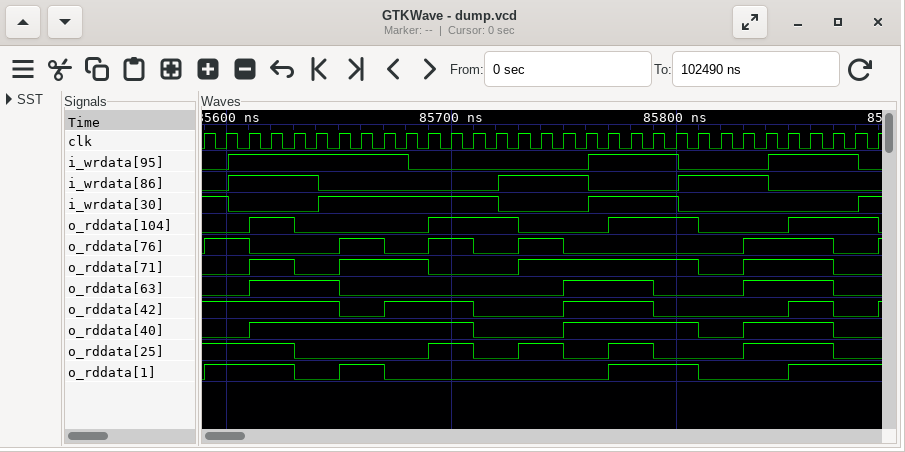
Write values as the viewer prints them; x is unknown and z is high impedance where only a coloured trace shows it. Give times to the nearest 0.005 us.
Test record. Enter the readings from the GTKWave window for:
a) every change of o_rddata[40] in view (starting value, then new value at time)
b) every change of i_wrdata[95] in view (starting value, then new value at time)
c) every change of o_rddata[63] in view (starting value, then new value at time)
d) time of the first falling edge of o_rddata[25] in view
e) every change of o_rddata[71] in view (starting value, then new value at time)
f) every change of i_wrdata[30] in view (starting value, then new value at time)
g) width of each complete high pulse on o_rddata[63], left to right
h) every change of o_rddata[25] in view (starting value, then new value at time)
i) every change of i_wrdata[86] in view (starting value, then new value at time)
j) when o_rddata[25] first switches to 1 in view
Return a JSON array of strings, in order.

["0, 1 at 85.61 us, 0 at 85.71 us, 1 at 85.75 us, 0 at 85.81 us, 1 at 85.83 us, 0 at 85.87 us", "0, 1 at 85.6 us, 0 at 85.68 us, 1 at 85.76 us, 0 at 85.8 us, 1 at 85.84 us, 0 at 85.88 us", "0, 1 at 85.61 us, 0 at 85.65 us, 1 at 85.75 us, 0 at 85.79 us, 1 at 85.83 us, 0 at 85.87 us", "85.63 us", "0, 1 at 85.61 us, 0 at 85.63 us, 1 at 85.65 us, 0 at 85.69 us, 1 at 85.73 us, 0 at 85.81 us, 1 at 85.83 us, 0 at 85.87 us", "1, 0 at 85.6 us, 1 at 85.64 us, 0 at 85.72 us, 1 at 85.76 us, 0 at 85.8 us, 1 at 85.88 us", "0.04 us, 0.04 us, 0.04 us", "1, 0 at 85.63 us, 1 at 85.69 us, 0 at 85.71 us, 1 at 85.73 us, 0 at 85.75 us, 1 at 85.77 us, 0 at 85.79 us, 1 at 85.83 us, 0 at 85.87 us", "0, 1 at 85.6 us, 0 at 85.64 us, 1 at 85.72 us, 0 at 85.76 us, 1 at 85.8 us, 0 at 85.84 us", "85.69 us"]
